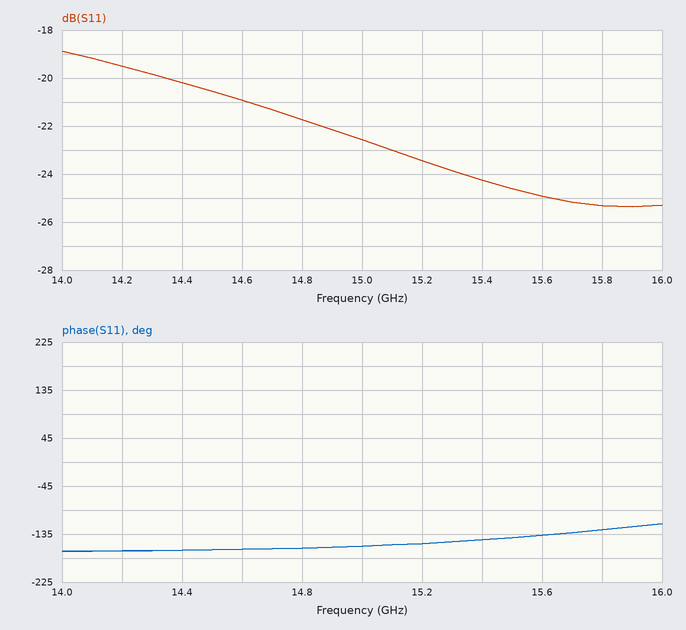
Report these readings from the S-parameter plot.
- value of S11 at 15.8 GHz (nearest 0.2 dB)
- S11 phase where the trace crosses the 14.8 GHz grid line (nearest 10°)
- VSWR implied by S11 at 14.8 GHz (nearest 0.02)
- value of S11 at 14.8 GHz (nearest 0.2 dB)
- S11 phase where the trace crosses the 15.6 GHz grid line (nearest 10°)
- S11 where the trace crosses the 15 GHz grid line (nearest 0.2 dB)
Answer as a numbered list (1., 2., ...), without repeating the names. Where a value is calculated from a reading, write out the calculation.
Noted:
1. -25.4 dB
2. -160°
3. |Γ| = 10^(-21.8/20) = 0.0813; VSWR = (1 + 0.0813)/(1 − 0.0813) ≈ 1.18
4. -21.8 dB
5. -140°
6. -22.6 dB
